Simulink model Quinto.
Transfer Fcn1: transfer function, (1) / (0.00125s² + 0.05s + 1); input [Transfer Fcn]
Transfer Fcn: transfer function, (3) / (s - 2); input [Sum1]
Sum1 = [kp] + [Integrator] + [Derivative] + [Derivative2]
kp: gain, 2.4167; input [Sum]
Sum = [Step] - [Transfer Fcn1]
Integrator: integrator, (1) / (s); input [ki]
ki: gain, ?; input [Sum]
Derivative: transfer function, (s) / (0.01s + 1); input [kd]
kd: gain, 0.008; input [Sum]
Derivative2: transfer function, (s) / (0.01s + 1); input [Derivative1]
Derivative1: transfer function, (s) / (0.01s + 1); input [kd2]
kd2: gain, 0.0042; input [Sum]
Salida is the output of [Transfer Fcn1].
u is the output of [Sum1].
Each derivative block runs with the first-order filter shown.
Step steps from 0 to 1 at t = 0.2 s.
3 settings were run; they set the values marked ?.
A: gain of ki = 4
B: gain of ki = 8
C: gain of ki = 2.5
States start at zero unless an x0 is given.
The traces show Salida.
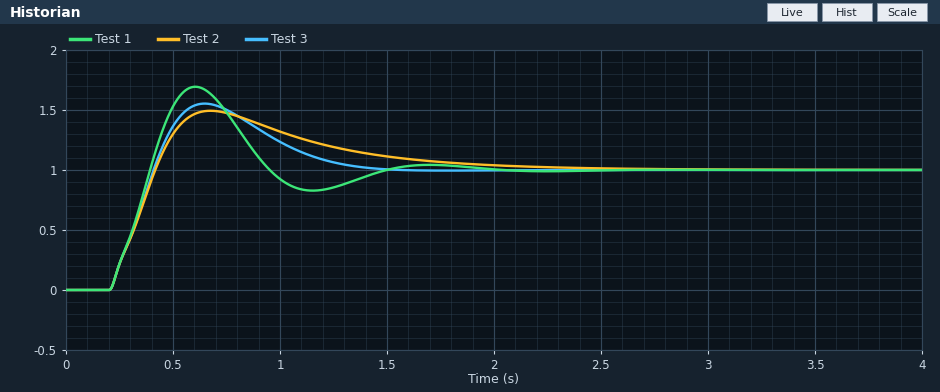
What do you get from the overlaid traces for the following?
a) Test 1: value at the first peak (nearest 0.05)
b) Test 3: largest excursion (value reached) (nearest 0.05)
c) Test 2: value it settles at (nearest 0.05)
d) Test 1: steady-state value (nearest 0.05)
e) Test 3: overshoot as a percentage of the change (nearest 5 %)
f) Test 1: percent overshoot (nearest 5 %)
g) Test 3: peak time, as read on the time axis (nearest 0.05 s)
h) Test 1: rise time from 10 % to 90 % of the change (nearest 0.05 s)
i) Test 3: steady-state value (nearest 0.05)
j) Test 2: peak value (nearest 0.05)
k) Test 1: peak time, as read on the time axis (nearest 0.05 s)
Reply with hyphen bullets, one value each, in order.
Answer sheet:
- 1.70
- 1.55
- 1.00
- 1.00
- 55 %
- 70 %
- 0.65 s
- 0.15 s
- 1.00
- 1.50
- 0.60 s
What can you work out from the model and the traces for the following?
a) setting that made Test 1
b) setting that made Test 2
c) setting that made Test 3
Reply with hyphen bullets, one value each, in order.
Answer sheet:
- B
- C
- A
